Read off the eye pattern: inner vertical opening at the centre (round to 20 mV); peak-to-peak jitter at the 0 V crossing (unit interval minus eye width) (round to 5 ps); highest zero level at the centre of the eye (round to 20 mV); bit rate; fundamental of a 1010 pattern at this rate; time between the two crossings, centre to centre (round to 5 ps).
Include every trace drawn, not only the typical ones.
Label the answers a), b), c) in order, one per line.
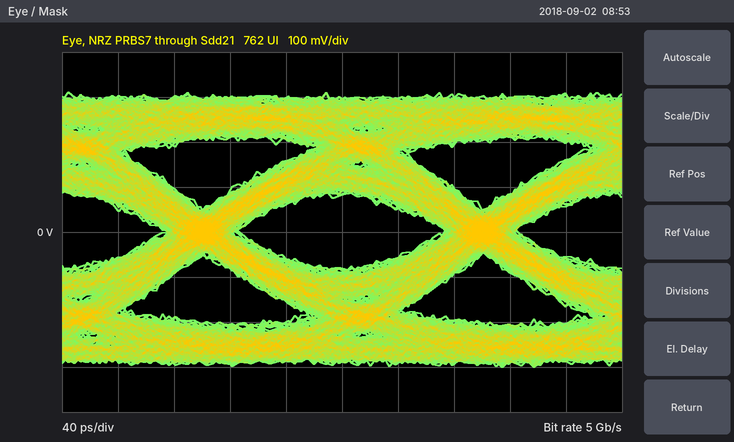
a) 160 mV
b) 55 ps
c) -80 mV
d) 5 Gb/s
e) 2.5 GHz
f) 200 ps
